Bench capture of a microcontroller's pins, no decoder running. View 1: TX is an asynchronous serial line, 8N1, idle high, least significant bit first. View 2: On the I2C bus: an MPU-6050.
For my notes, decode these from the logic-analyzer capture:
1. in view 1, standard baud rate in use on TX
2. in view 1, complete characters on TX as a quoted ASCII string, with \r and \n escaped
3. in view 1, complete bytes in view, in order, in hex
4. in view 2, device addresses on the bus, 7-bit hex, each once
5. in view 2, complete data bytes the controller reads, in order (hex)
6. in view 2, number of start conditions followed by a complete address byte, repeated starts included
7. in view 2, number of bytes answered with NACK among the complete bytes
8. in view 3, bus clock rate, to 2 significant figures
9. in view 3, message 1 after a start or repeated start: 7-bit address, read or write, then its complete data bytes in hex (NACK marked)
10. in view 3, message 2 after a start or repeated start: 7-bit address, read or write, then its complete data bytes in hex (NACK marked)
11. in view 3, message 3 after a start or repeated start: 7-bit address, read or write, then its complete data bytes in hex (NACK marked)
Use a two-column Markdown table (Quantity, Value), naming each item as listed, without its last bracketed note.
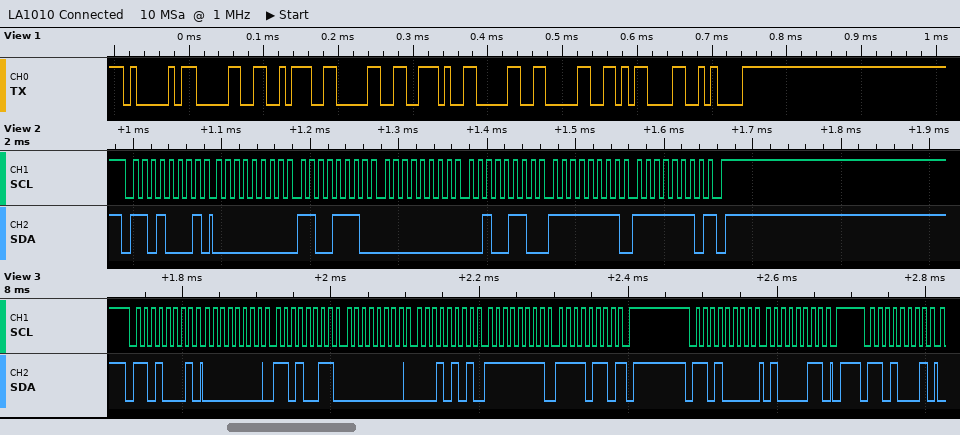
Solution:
| Quantity | Value |
|---|---|
| in view 1, standard baud rate in use on TX | 115200 baud |
| in view 1, complete characters on TX as a quoted ASCII string, with \r and \n escaped | "A0:0.00\r\n" |
| in view 1, complete bytes in view, in order, in hex | 0x41 0x30 0x3A 0x30 0x2E 0x30 0x30 0x0D 0x0A |
| in view 2, device addresses on the bus, 7-bit hex, each once | 0x68 |
| in view 2, complete data bytes the controller reads, in order | 00 CE 00 26 FF FE |
| in view 2, number of start conditions followed by a complete address byte, repeated starts included | 1 |
| in view 2, number of bytes answered with NACK among the complete bytes | 1 |
| in view 3, bus clock rate, to 2 significant figures | 100 kHz |
| in view 3, message 1 after a start or repeated start: 7-bit address, read or write, then its complete data bytes in hex | 0x68 read: 00 D3 00 15 FF F6 NACK |
| in view 3, message 2 after a start or repeated start: 7-bit address, read or write, then its complete data bytes in hex | 0x68 write: 43 |
| in view 3, message 3 after a start or repeated start: 7-bit address, read or write, then its complete data bytes in hex | 0x68 read |
